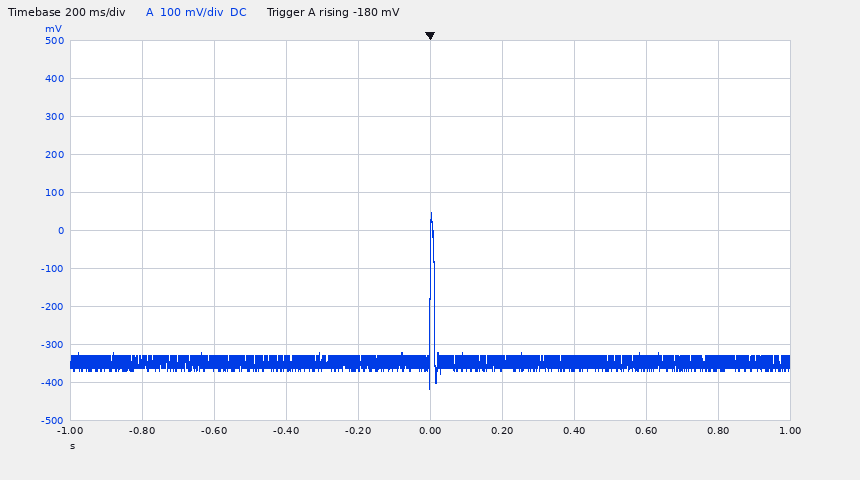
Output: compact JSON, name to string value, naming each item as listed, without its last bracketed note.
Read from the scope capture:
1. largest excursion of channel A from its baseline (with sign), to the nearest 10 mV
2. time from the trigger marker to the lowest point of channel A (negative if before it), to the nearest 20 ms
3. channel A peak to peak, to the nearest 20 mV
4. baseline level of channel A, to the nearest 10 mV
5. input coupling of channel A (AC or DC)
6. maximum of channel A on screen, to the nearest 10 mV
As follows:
{"largest excursion of channel A from its baseline (with sign), to the nearest 10 mV": "+390 mV", "time from the trigger marker to the lowest point of channel A (negative if before it), to the nearest 20 ms": "0 ms", "channel A peak to peak, to the nearest 20 mV": "460 mV", "baseline level of channel A, to the nearest 10 mV": "-340 mV", "input coupling of channel A": "DC", "maximum of channel A on screen, to the nearest 10 mV": "50 mV"}
